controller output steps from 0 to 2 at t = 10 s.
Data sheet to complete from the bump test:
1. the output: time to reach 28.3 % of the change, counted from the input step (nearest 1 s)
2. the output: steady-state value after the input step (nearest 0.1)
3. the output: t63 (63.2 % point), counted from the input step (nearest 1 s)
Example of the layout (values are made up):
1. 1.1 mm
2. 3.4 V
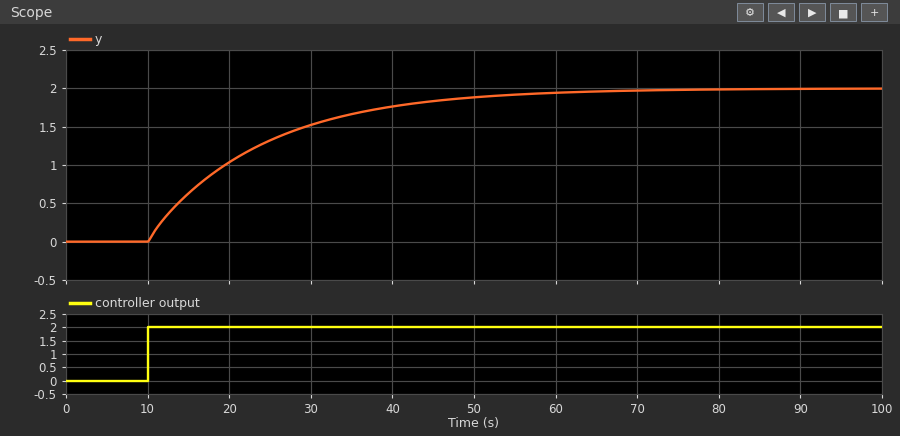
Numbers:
1. 4 s
2. 2.0
3. 14 s
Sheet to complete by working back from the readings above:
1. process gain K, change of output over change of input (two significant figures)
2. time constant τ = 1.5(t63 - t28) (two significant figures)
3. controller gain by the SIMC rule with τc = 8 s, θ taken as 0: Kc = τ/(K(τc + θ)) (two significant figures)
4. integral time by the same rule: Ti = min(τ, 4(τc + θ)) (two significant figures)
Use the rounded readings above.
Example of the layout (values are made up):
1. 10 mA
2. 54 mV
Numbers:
1. 1.0
2. 15 s
3. 1.9
4. 15 s
